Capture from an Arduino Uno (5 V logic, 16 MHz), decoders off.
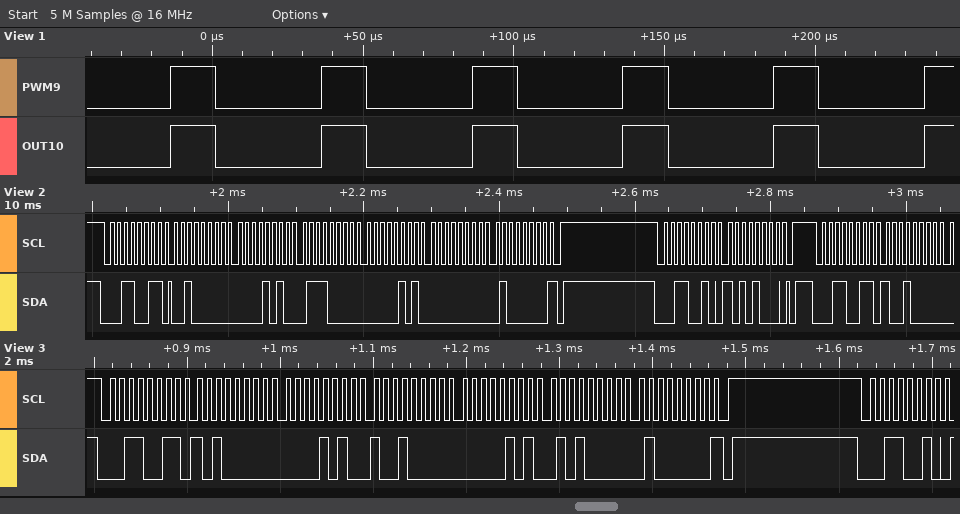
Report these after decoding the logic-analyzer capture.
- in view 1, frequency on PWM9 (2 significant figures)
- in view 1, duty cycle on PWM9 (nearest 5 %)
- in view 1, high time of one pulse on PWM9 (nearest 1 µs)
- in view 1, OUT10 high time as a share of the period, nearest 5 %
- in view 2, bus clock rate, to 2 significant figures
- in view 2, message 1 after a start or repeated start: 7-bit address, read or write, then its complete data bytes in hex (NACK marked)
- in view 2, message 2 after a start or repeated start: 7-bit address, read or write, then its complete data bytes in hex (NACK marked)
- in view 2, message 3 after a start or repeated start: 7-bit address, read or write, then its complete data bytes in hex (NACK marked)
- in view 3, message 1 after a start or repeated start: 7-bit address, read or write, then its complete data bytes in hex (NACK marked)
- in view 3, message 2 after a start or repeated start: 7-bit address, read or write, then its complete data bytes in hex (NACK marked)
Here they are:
20 kHz
30 %
15 µs
30 %
100 kHz
0x19 read: 20 0A 70 05 00 40 NACK
0x19 write: A8
0x19 read: 90
0x19 read: A0 0A 90 05 50 40 NACK
0x19 write
